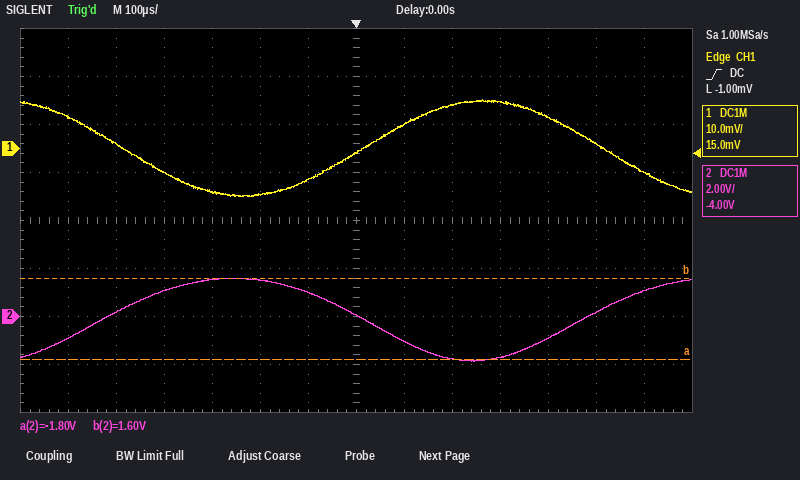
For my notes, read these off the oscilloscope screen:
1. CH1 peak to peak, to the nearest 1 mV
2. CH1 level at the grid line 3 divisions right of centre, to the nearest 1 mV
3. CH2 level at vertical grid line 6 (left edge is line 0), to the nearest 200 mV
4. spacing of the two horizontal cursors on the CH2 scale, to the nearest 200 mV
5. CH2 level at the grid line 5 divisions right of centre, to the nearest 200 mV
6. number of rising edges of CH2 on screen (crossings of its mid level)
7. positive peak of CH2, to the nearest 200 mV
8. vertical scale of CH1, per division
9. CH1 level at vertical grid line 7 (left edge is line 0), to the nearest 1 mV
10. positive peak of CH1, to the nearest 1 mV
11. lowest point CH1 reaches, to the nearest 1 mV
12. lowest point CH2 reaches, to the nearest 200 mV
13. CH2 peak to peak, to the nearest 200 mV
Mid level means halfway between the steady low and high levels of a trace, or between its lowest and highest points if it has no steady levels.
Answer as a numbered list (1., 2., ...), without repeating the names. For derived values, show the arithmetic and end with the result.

1. 10 mV − (-10 mV) = 20 mV
2. 10 mV
3. 1.0 V
4. 3.4 V
5. 200 mV
6. 2
7. 1.6 V
8. 10 mV
9. -1 mV
10. 10 mV
11. -10 mV
12. -1.8 V
13. 1.6 V − (-1.8 V) = 3.4 V
